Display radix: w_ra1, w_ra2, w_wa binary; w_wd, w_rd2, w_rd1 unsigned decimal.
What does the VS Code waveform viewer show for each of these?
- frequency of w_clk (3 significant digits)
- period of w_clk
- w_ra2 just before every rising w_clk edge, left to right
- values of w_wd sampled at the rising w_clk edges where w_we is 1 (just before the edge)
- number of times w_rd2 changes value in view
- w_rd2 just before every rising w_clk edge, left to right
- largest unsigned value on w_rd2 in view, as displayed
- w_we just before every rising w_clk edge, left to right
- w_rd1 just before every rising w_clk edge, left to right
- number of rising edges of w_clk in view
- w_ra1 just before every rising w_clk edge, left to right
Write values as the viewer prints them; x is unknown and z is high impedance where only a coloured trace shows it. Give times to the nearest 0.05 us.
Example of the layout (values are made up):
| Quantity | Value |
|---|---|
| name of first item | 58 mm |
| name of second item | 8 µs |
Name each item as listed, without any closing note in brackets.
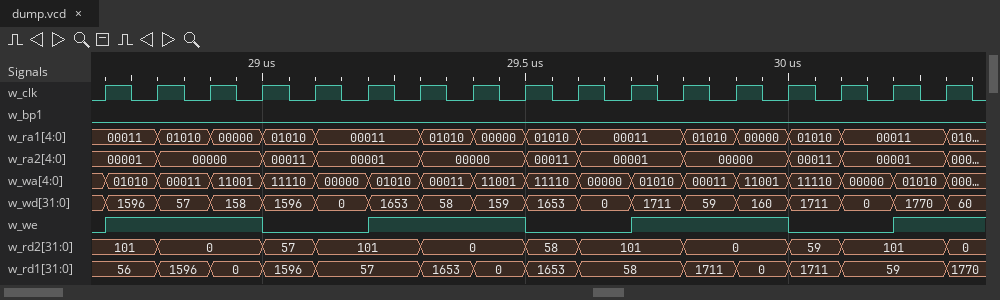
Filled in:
| Quantity | Value |
|---|---|
| frequency of w_clk | 10.0 MHz |
| period of w_clk | 0.1 us |
| w_ra2 just before every rising w_clk edge, left to right | 00001, 00001, 00000, 00000, 00011, 00001, 00001, 00000, 00000, 00011, 00001, 00001, 00000, 00000, 00011, 00001, 00001 |
| values of w_wd sampled at the rising w_clk edges where w_we is 1 | 1596, 57, 158, 1653, 58, 159, 1711, 59, 160, 1770 |
| number of times w_rd2 changes value in view | 10 |
| w_rd2 just before every rising w_clk edge, left to right | 101, 101, 0, 0, 57, 101, 101, 0, 0, 58, 101, 101, 0, 0, 59, 101, 101 |
| largest unsigned value on w_rd2 in view, as displayed | 101 |
| w_we just before every rising w_clk edge, left to right | 0 1 1 1 0 0 1 1 1 0 0 1 1 1 0 0 1 |
| w_rd1 just before every rising w_clk edge, left to right | 56, 56, 1596, 0, 1596, 57, 57, 1653, 0, 1653, 58, 58, 1711, 0, 1711, 59, 59 |
| number of rising edges of w_clk in view | 17 |
| w_ra1 just before every rising w_clk edge, left to right | 00011, 00011, 01010, 00000, 01010, 00011, 00011, 01010, 00000, 01010, 00011, 00011, 01010, 00000, 01010, 00011, 00011 |
